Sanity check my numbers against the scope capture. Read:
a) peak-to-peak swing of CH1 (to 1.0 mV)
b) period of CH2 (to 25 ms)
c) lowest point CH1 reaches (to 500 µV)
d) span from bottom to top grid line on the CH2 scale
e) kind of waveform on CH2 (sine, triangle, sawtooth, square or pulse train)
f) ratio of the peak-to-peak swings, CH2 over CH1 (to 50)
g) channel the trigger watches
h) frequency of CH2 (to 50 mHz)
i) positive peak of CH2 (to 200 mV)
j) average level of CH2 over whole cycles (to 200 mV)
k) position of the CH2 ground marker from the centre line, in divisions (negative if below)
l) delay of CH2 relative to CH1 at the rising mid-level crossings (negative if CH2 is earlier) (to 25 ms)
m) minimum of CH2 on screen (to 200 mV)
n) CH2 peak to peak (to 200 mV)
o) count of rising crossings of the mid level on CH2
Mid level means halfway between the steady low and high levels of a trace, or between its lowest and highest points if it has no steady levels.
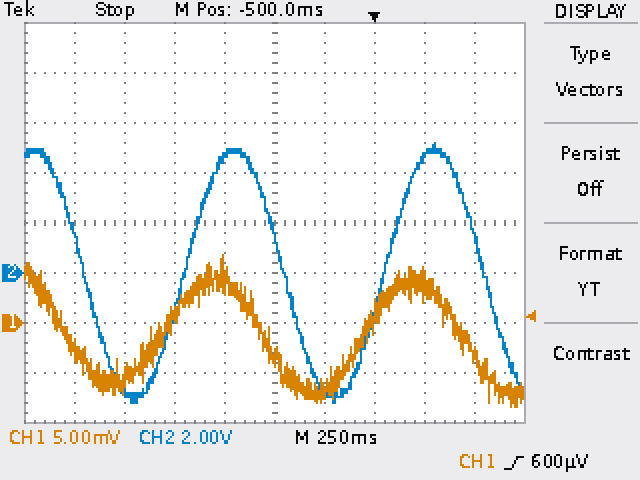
15.0 mV
1.000 s
-8.5 mV
16 V
sine
700
CH1
1.00 Hz
5.2 V
0.0 V
-1.0 div
+100 ms
-5.2 V
10.4 V
2
